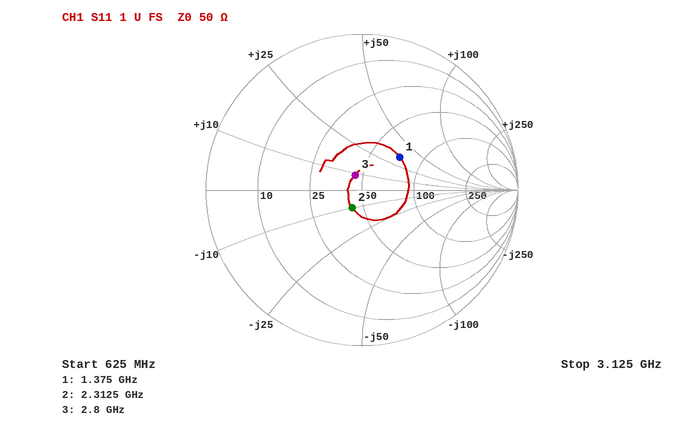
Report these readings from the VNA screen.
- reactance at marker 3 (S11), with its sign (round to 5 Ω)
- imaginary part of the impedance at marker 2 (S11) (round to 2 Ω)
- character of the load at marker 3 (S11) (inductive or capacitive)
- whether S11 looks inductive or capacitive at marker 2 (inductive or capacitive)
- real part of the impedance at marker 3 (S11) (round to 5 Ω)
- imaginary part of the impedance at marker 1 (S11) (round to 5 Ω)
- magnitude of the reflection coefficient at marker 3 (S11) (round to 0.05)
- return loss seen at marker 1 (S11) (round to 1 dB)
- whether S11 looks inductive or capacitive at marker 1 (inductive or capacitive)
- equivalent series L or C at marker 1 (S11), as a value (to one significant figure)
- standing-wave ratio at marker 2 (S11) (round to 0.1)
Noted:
+10 Ω
-10 Ω
inductive
capacitive
45 Ω
+35 Ω
0.10
10 dB
inductive
4 nH
1.3
